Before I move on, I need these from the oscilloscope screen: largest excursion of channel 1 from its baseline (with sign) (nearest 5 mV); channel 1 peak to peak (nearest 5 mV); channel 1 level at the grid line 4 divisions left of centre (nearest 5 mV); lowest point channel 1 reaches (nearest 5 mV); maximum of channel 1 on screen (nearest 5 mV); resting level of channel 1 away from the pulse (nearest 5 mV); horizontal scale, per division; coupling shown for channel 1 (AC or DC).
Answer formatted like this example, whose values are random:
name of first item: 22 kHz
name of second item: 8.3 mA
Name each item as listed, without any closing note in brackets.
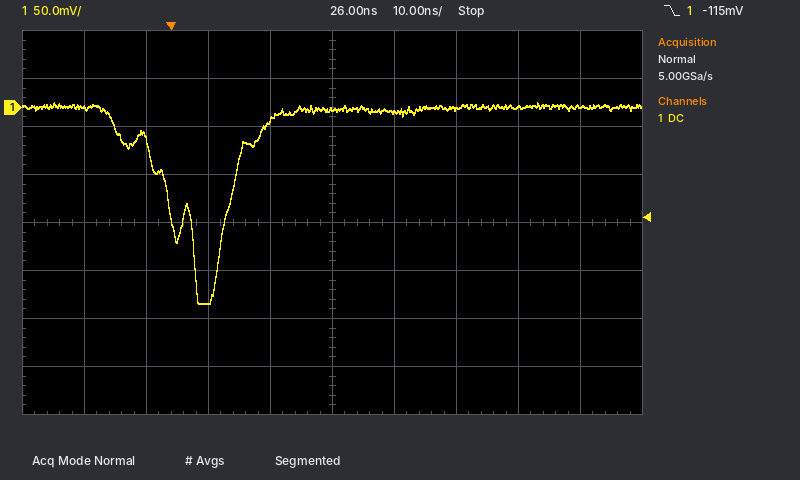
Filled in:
largest excursion of channel 1 from its baseline (with sign): -205 mV
channel 1 peak to peak: 210 mV
channel 1 level at the grid line 4 divisions left of centre: 0 mV
lowest point channel 1 reaches: -205 mV
maximum of channel 1 on screen: 5 mV
resting level of channel 1 away from the pulse: 0 mV
horizontal scale, per division: 10 ns
coupling shown for channel 1: DC
